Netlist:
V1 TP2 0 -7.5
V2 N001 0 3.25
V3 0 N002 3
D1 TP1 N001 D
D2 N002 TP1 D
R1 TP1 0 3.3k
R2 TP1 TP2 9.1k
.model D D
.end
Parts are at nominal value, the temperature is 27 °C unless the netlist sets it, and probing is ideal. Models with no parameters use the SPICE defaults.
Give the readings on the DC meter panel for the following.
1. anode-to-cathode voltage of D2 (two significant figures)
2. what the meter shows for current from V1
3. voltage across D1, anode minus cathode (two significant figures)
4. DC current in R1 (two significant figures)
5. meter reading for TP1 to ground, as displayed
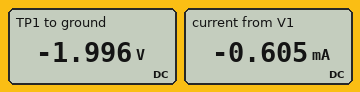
-1.0 V
-0.605 mA
-5.2 V
600 µA
-1.996 V
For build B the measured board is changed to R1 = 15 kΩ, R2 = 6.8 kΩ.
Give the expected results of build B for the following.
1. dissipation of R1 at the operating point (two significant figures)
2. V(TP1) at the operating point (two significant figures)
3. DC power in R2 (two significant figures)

880 µW
-3.6 V
2.2 mW
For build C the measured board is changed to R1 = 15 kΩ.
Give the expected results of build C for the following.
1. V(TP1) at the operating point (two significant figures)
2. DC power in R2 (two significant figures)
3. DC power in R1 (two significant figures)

-3.6 V
1.7 mW
870 µW
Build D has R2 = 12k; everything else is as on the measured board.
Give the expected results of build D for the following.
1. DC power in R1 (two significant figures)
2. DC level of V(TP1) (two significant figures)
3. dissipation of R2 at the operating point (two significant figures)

790 µW
-1.6 V
2.9 mW
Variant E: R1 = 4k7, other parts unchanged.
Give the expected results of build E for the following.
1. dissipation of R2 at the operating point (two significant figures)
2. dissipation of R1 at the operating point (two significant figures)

2.7 mW
1.4 mW
